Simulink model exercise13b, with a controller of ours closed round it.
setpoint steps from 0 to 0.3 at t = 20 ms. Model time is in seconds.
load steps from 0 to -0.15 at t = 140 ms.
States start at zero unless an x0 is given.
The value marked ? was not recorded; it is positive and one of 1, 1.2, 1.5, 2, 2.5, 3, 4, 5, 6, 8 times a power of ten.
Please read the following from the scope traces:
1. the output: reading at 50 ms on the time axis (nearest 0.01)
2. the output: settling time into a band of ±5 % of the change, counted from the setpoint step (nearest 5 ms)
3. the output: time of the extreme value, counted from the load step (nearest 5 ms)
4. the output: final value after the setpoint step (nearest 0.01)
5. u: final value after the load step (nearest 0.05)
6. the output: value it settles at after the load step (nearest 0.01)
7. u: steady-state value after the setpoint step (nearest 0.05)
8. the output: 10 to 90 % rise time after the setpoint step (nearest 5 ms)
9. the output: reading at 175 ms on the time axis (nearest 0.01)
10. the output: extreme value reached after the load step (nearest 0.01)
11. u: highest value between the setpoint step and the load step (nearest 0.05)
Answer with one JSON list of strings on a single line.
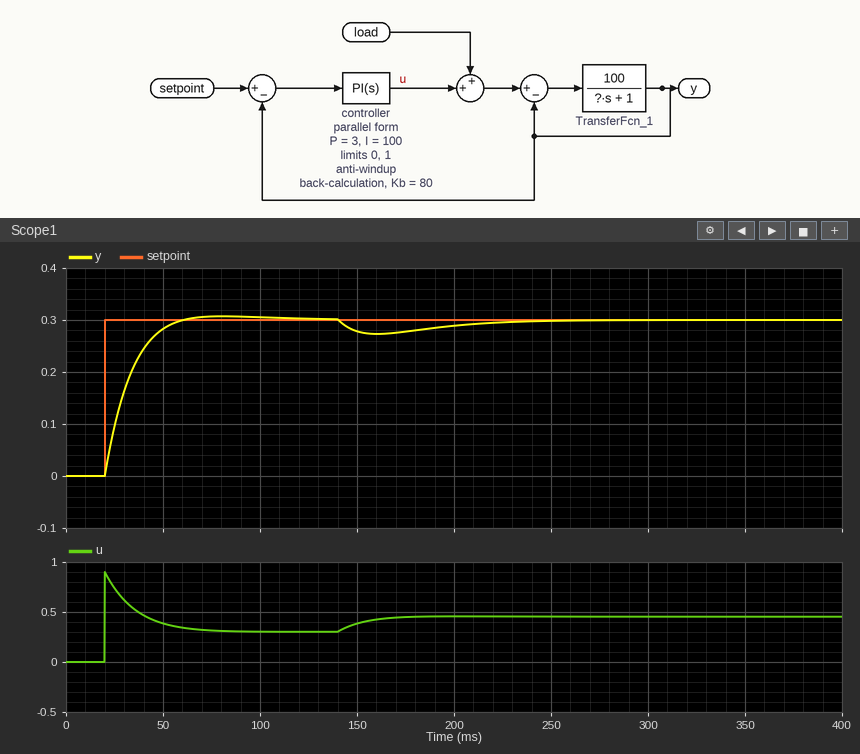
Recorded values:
["0.28", "30 ms", "20 ms", "0.30", "0.45", "0.30", "0.30", "25 ms", "0.28", "0.27", "0.90"]
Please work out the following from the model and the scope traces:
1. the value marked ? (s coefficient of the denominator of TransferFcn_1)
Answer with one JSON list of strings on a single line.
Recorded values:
["4"]
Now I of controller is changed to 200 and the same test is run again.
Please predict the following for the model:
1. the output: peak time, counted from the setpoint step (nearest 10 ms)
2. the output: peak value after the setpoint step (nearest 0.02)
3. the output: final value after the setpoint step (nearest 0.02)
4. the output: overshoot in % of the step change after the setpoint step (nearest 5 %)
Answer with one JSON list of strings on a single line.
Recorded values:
["40 ms", "0.34", "0.30", "10 %"]
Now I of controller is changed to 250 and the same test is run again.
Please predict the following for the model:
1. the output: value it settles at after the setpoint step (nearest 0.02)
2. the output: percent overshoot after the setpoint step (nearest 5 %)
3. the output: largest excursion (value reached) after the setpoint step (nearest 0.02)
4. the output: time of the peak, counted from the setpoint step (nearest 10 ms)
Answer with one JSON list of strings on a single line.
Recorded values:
["0.30", "15 %", "0.34", "30 ms"]
